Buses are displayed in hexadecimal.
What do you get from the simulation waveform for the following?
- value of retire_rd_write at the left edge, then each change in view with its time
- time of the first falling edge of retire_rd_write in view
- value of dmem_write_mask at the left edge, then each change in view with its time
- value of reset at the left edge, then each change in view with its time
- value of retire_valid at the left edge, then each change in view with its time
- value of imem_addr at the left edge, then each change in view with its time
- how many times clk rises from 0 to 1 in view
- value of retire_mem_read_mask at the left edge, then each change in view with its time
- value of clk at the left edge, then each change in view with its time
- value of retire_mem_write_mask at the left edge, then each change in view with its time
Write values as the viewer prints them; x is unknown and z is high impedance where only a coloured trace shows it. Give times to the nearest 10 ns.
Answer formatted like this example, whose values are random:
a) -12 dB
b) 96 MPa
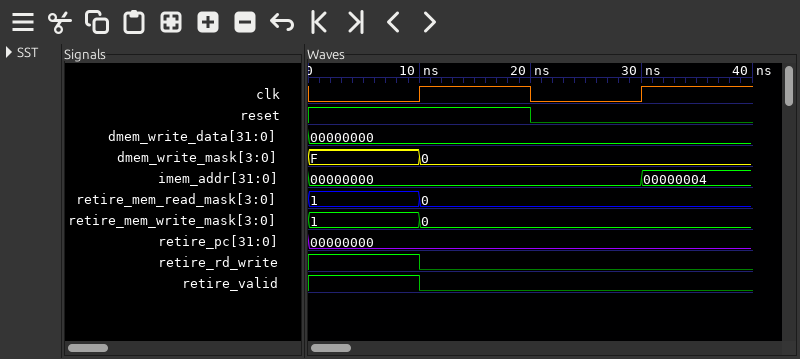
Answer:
a) 1, 0 at 10 ns
b) 10 ns
c) F, 0 at 10 ns
d) 1, 0 at 20 ns
e) 1, 0 at 10 ns
f) 00000000, 00000004 at 30 ns
g) 2
h) 1, 0 at 10 ns
i) 0, 1 at 10 ns, 0 at 20 ns, 1 at 30 ns
j) 1, 0 at 10 ns
